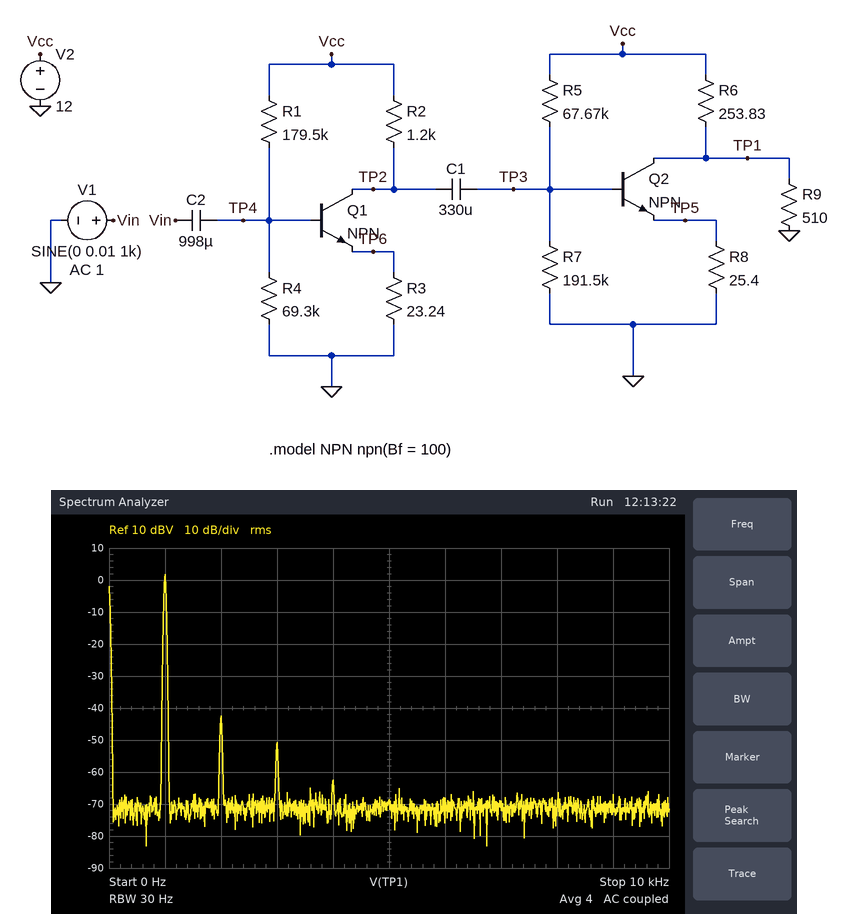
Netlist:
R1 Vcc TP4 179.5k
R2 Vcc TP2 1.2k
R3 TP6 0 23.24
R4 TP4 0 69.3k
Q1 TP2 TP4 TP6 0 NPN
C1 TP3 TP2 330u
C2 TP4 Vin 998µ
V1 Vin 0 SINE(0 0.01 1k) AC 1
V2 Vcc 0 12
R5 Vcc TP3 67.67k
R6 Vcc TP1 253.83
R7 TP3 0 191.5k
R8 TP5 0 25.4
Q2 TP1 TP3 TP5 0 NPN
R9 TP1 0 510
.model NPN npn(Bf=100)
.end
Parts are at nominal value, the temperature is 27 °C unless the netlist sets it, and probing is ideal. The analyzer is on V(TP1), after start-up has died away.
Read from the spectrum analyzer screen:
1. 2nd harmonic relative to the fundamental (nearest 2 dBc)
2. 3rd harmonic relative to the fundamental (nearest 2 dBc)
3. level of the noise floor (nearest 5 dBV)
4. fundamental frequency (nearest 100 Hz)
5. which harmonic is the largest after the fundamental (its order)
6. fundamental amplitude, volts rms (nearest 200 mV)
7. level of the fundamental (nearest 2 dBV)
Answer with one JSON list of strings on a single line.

["-44 dBc", "-52 dBc", "-70 dBV", "1.0 kHz", "2", "1.2 V", "2 dBV"]
